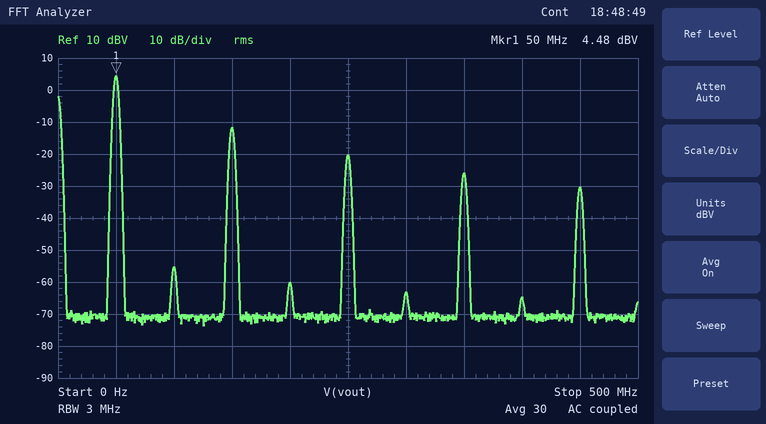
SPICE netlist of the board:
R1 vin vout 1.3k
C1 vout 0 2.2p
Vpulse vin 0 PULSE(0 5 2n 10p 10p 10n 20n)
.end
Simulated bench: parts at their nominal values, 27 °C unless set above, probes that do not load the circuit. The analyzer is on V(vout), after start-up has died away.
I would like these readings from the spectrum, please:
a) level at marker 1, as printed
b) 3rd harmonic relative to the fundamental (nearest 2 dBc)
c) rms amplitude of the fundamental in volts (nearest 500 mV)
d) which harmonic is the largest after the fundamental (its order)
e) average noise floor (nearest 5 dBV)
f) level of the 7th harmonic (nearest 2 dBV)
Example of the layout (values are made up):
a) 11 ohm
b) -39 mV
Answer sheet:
a) 4.48 dBV
b) -16 dBc
c) 1.5 V
d) 3
e) -70 dBV
f) -26 dBV
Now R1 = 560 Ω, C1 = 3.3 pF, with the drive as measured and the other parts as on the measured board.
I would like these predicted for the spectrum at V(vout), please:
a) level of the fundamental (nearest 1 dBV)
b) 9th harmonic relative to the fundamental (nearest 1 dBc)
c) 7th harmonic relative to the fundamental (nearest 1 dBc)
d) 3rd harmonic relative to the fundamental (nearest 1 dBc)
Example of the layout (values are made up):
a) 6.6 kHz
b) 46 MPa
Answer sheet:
a) 6 dBV
b) -32 dBc
c) -28 dBc
d) -14 dBc
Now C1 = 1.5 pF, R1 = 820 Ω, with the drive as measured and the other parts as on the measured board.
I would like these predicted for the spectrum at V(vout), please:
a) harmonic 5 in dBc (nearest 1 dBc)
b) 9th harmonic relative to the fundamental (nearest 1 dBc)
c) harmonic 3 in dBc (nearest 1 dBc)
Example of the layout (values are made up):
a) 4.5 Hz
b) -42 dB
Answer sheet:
a) -20 dBc
b) -30 dBc
c) -13 dBc
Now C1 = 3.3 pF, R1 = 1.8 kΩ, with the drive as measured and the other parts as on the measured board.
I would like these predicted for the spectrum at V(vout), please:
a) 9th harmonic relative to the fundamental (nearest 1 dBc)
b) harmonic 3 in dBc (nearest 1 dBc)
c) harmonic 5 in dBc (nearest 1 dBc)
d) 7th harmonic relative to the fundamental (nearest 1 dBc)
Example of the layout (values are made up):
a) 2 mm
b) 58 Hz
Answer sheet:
a) -37 dBc
b) -18 dBc
c) -27 dBc
d) -33 dBc
